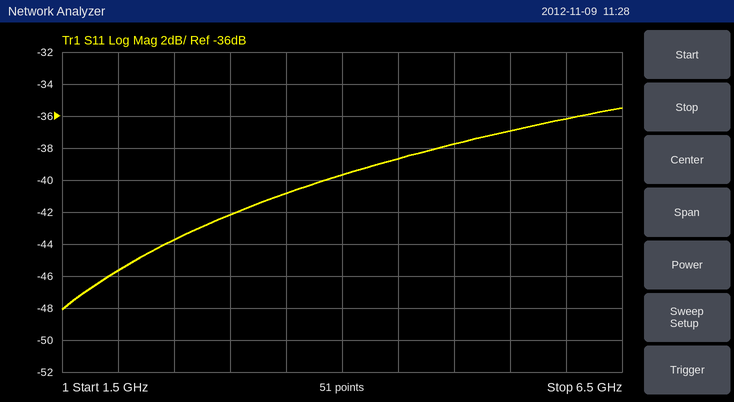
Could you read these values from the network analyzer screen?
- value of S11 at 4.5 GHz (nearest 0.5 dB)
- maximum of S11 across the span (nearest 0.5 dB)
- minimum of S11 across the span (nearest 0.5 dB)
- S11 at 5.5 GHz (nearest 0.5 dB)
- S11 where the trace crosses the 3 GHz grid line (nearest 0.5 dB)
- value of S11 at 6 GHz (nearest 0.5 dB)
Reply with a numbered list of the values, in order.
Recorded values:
1. -38.5 dB
2. -35.5 dB
3. -48.0 dB
4. -37.0 dB
5. -42.0 dB
6. -36.0 dB
